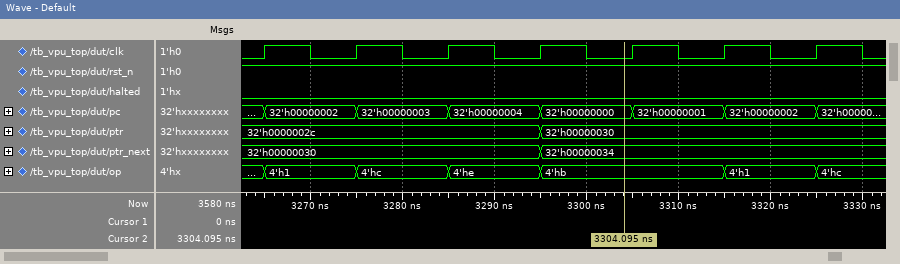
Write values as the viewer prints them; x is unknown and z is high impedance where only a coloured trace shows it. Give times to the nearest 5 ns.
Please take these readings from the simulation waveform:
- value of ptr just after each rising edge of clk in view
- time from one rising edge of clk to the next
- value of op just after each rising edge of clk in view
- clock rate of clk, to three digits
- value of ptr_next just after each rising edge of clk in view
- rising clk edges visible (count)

32'h0000002c, 32'h0000002c, 32'h0000002c, 32'h00000030, 32'h00000030, 32'h00000030, 32'h00000030
10 ns
4'h1, 4'hc, 4'he, 4'hb, 4'hb, 4'h1, 4'hc
100 MHz
32'h00000030, 32'h00000030, 32'h00000030, 32'h00000034, 32'h00000034, 32'h00000034, 32'h00000034
7
